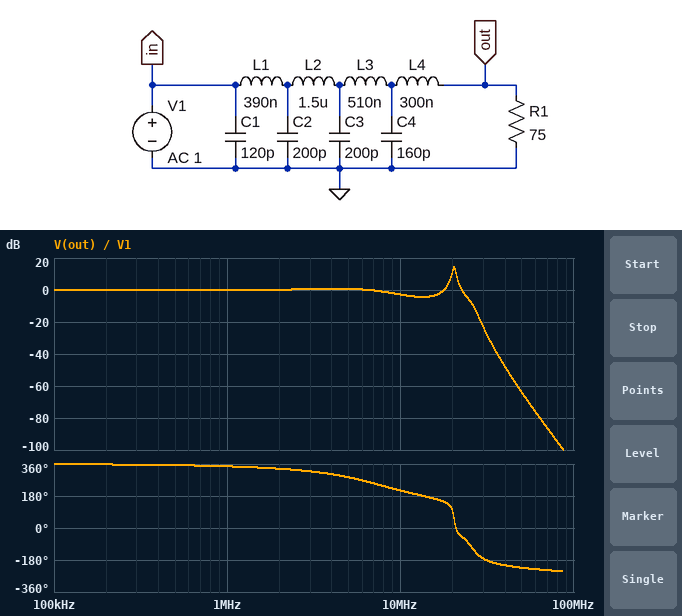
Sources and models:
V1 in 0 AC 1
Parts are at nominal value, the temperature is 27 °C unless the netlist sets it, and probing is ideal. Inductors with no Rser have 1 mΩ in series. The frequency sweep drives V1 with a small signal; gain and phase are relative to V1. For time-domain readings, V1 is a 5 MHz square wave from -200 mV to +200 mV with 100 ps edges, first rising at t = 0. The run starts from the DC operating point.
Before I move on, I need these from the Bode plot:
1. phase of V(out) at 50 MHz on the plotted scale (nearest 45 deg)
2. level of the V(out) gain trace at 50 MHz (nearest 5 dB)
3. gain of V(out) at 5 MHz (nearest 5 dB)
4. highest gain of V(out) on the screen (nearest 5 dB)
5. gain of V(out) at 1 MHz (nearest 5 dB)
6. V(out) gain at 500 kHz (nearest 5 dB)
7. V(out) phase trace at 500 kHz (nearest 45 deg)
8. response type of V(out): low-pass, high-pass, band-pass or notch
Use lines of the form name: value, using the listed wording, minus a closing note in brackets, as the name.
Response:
phase of V(out) at 50 MHz on the plotted scale: -225 deg
level of the V(out) gain trace at 50 MHz: -65 dB
gain of V(out) at 5 MHz: 0 dB
highest gain of V(out) on the screen: 15 dB
gain of V(out) at 1 MHz: 0 dB
V(out) gain at 500 kHz: 0 dB
V(out) phase trace at 500 kHz: 360 deg
response type of V(out): low-pass, high-pass, band-pass or notch: band-pass
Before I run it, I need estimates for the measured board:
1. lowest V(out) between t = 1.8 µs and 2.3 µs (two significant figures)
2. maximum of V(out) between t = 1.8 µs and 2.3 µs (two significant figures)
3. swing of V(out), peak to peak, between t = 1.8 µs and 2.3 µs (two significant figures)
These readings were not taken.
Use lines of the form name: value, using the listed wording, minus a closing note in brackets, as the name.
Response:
lowest V(out) between t = 1.8 µs and 2.3 µs: -280 mV
maximum of V(out) between t = 1.8 µs and 2.3 µs: 280 mV
swing of V(out), peak to peak, between t = 1.8 µs and 2.3 µs: 570 mV
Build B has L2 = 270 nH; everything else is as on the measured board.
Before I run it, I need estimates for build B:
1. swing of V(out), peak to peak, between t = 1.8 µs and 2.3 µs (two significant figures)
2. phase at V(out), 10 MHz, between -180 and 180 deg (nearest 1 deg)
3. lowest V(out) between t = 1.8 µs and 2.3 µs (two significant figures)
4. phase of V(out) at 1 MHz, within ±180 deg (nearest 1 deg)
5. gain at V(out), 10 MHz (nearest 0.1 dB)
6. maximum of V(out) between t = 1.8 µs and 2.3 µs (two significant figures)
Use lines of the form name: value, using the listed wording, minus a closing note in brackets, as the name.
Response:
swing of V(out), peak to peak, between t = 1.8 µs and 2.3 µs: 700 mV
phase at V(out), 10 MHz, between -180 and 180 deg: -111 deg
lowest V(out) between t = 1.8 µs and 2.3 µs: -350 mV
phase of V(out) at 1 MHz, within ±180 deg: -7 deg
gain at V(out), 10 MHz: 4.9 dB
maximum of V(out) between t = 1.8 µs and 2.3 µs: 350 mV
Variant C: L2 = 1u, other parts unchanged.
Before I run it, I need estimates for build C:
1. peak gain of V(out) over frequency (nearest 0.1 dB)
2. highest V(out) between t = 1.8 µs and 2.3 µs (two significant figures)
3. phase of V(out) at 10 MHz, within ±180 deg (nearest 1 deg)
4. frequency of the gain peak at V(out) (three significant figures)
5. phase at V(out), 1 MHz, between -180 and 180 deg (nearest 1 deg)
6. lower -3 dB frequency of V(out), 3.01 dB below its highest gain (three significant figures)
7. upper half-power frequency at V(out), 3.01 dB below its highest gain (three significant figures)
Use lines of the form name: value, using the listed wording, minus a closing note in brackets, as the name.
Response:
peak gain of V(out) over frequency: 10.1 dB
highest V(out) between t = 1.8 µs and 2.3 µs: 310 mV
phase of V(out) at 10 MHz, within ±180 deg: -141 deg
frequency of the gain peak at V(out): 21.3 MHz
phase at V(out), 1 MHz, between -180 and 180 deg: -11 deg
lower -3 dB frequency of V(out), 3.01 dB below its highest gain: 20.2 MHz
upper half-power frequency at V(out), 3.01 dB below its highest gain: 22.4 MHz
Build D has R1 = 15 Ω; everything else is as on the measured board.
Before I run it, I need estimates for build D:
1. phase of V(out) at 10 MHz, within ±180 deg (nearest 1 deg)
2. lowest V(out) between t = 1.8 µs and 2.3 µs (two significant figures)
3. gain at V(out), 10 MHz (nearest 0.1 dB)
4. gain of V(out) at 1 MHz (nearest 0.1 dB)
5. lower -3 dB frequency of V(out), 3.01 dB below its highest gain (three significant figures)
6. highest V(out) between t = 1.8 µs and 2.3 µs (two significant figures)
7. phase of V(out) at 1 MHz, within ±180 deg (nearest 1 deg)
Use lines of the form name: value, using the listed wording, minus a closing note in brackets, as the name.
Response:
phase of V(out) at 10 MHz, within ±180 deg: -109 deg
lowest V(out) between t = 1.8 µs and 2.3 µs: -77 mV
gain at V(out), 10 MHz: -11.5 dB
gain of V(out) at 1 MHz: -3.4 dB
lower -3 dB frequency of V(out), 3.01 dB below its highest gain: 20.6 MHz
highest V(out) between t = 1.8 µs and 2.3 µs: 77 mV
phase of V(out) at 1 MHz, within ±180 deg: -49 deg
